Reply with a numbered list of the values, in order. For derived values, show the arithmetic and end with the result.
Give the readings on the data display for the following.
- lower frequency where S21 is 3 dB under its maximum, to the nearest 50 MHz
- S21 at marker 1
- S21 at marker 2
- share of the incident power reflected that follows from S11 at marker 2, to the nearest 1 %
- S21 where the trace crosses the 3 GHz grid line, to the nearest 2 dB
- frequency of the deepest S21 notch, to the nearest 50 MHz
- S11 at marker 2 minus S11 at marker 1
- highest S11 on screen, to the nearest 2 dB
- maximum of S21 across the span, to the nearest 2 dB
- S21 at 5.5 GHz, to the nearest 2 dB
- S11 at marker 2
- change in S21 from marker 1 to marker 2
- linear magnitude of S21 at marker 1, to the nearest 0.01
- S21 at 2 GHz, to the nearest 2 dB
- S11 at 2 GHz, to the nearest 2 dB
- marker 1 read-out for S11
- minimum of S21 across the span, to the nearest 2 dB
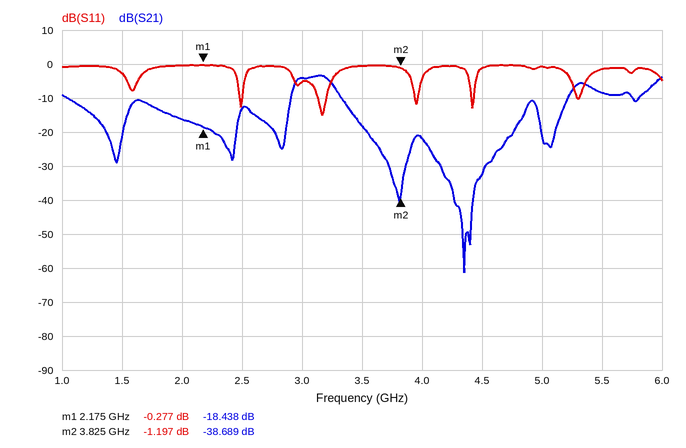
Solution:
1. 2.95 GHz
2. -18.438 dB
3. -38.689 dB
4. 10^(-1.197/10) ≈ 76 %
5. -4 dB
6. 4.35 GHz
7. -1.197 − (-0.277) = -0.920 dB
8. 0 dB
9. -4 dB
10. -8 dB
11. -1.197 dB
12. -38.689 − (-18.438) = -20.251 dB
13. 10^(-18.438/20) ≈ 0.12
14. -16 dB
15. 0 dB
16. -0.277 dB
17. -62 dB
